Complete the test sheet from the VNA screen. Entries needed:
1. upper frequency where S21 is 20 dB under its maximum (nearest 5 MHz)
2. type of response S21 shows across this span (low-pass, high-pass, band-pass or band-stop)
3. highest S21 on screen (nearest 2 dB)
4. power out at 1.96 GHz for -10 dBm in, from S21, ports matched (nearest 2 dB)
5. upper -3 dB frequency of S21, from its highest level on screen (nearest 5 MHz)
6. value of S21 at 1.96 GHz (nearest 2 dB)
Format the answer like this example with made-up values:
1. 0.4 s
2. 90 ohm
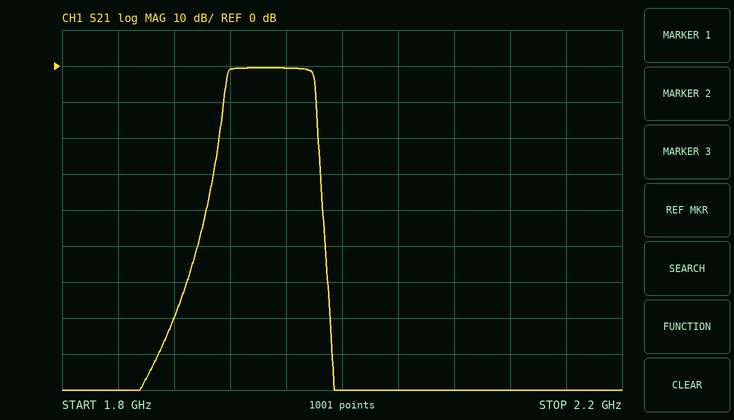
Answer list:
1. 1.985 GHz
2. band-pass
3. 0 dB
4. -10 dBm
5. 1.980 GHz
6. 0 dB
